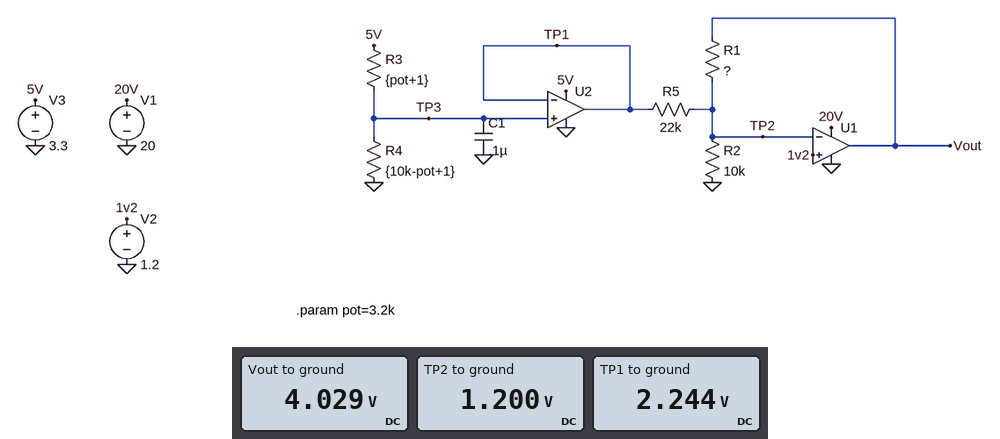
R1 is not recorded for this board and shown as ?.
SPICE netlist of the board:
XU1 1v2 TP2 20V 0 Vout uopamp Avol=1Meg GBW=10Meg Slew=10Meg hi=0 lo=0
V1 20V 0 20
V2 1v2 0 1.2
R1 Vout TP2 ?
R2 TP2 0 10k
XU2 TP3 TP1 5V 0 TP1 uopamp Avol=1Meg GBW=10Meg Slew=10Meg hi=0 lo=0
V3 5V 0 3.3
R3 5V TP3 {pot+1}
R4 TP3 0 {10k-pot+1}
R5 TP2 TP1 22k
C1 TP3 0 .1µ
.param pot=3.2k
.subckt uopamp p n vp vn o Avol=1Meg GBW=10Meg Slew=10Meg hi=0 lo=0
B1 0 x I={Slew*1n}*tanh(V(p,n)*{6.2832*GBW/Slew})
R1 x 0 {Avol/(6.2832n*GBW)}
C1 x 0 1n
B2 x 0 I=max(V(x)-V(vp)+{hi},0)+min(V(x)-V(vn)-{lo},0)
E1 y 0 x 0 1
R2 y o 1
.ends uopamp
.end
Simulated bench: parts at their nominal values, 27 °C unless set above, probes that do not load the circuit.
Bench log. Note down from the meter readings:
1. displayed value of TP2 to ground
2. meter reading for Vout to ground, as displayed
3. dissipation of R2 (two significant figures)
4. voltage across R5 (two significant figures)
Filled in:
1.200 V
4.029 V
140 µW
1.0 V
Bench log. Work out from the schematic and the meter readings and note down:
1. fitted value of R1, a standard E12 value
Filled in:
39 kΩ
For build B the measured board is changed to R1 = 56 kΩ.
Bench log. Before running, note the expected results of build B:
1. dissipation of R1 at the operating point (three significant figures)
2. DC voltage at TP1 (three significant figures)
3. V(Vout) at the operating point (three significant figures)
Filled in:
295 µW
2.24 V
5.26 V
